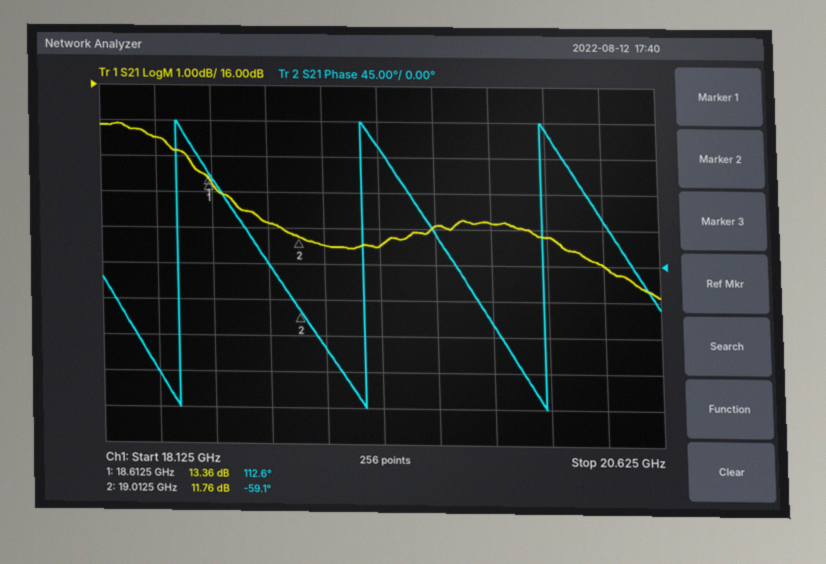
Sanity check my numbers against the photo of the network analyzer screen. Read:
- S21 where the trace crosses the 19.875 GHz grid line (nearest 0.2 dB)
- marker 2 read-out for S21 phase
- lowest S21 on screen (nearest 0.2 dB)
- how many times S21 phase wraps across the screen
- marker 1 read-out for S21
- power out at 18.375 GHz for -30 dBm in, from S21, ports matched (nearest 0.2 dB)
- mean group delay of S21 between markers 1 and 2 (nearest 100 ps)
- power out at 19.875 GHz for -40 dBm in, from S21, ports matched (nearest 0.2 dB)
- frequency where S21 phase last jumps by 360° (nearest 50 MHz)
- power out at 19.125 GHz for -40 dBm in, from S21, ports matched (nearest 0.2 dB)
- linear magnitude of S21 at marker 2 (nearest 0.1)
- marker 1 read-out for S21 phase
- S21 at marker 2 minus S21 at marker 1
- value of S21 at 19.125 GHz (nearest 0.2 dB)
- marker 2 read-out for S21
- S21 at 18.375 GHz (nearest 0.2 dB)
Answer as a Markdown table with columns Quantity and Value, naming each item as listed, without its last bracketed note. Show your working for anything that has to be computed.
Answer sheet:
| Quantity | Value |
|---|---|
| S21 where the trace crosses the 19.875 GHz grid line | 12.2 dB |
| marker 2 read-out for S21 phase | -59.1° |
| lowest S21 on screen | 10.2 dB |
| how many times S21 phase wraps across the screen | 3 |
| marker 1 read-out for S21 | 13.36 dB |
| power out at 18.375 GHz for -30 dBm in, from S21, ports matched | -30 dBm + (14.6 dB) = -15.4 dBm |
| mean group delay of S21 between markers 1 and 2 | −(-59.1° − (112.6°))/(360° × 400 MHz) ≈ 1.2 ns |
| power out at 19.875 GHz for -40 dBm in, from S21, ports matched | -40 dBm + (12.2 dB) = -27.8 dBm |
| frequency where S21 phase last jumps by 360° | 20.10 GHz |
| power out at 19.125 GHz for -40 dBm in, from S21, ports matched | -40 dBm + (11.6 dB) = -28.4 dBm |
| linear magnitude of S21 at marker 2 | 10^(11.76/20) ≈ 3.9 |
| marker 1 read-out for S21 phase | 112.6° |
| S21 at marker 2 minus S21 at marker 1 | 11.76 − (13.36) = -1.60 dB |
| value of S21 at 19.125 GHz | 11.6 dB |
| marker 2 read-out for S21 | 11.76 dB |
| S21 at 18.375 GHz | 14.6 dB |
